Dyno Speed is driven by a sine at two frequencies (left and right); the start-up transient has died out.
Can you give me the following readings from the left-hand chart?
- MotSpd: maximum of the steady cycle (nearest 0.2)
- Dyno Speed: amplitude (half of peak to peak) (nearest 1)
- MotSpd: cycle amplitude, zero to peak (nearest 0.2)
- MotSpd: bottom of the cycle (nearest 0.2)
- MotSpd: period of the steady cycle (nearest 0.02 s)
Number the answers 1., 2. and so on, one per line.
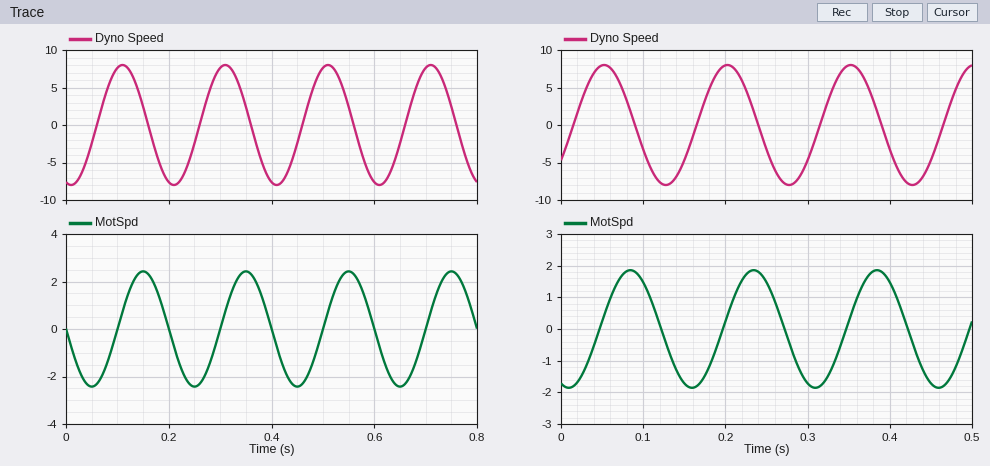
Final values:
1. 2.4
2. 8
3. 2.4
4. -2.4
5. 0.20 s
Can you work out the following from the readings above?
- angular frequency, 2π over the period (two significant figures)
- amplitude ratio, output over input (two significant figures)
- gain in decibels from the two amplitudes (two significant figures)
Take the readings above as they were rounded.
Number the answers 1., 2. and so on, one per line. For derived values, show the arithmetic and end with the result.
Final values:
1. 2π / 0.2 = 31 rad/s
2. 2.4 / 8 = 0.30
3. 20 log10(2.4 / 8) = -10 dB
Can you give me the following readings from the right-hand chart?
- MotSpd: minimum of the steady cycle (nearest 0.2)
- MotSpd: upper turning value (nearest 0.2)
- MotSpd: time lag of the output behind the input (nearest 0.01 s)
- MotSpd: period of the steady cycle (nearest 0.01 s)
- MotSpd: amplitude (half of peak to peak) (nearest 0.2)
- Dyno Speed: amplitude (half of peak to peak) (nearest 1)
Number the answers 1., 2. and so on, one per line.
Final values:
1. -1.8
2. 1.8
3. 0.03 s
4. 0.15 s
5. 1.8
6. 8
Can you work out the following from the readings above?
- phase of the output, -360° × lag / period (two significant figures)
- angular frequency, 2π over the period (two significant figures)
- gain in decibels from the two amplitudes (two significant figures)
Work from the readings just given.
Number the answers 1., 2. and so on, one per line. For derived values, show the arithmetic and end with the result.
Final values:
1. -360 × 0.03 / 0.15 = -72°
2. 2π / 0.15 = 42 rad/s
3. 20 log10(1.8 / 8) = -13 dB
